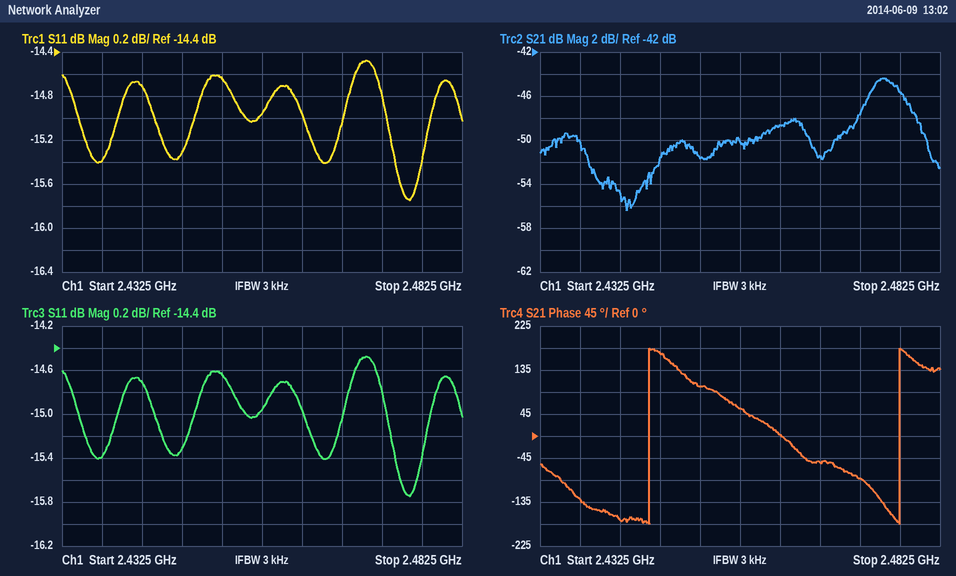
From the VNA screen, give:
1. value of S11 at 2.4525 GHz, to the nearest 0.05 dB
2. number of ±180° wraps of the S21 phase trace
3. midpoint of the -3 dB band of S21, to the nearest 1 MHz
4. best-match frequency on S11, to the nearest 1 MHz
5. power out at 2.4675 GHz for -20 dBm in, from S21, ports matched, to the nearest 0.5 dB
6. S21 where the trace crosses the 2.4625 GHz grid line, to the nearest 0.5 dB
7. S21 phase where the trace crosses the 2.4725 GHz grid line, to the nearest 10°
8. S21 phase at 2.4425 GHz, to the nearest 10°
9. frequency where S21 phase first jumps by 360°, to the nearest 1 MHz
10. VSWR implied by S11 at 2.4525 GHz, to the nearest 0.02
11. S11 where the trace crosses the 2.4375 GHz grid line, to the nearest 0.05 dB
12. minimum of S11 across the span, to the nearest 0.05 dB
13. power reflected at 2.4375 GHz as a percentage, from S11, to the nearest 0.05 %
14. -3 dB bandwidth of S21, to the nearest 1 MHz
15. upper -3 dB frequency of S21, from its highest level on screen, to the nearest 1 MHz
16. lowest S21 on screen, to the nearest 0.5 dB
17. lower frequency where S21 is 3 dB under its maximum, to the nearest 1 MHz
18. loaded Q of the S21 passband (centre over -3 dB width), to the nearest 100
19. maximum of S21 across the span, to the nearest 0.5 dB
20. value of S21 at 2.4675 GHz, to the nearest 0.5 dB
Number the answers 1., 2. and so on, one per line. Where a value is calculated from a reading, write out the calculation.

1. -14.65 dB
2. 2
3. 2.476 GHz
4. 2.476 GHz
5. -20 dBm + (-51.5 dB) = -71.5 dBm
6. -48.5 dB
7. -90°
8. -170°
9. 2.446 GHz
10. |Γ| = 10^(-14.65/20) = 0.1851; VSWR = (1 + 0.1851)/(1 − 0.1851) ≈ 1.45, so 1.46 to the nearest 0.02
11. -15.40 dB
12. -15.75 dB
13. 10^(-15.4/10) ≈ 2.88 %, so 2.90 % to the nearest 0.05 %
14. 2.479 GHz − 2.473 GHz = 6 MHz
15. 2.479 GHz
16. -56.5 dB
17. 2.473 GHz
18. 2.476 GHz / 6 MHz ≈ 413, so 400 to the nearest 100
19. -44.5 dB
20. -51.5 dB
